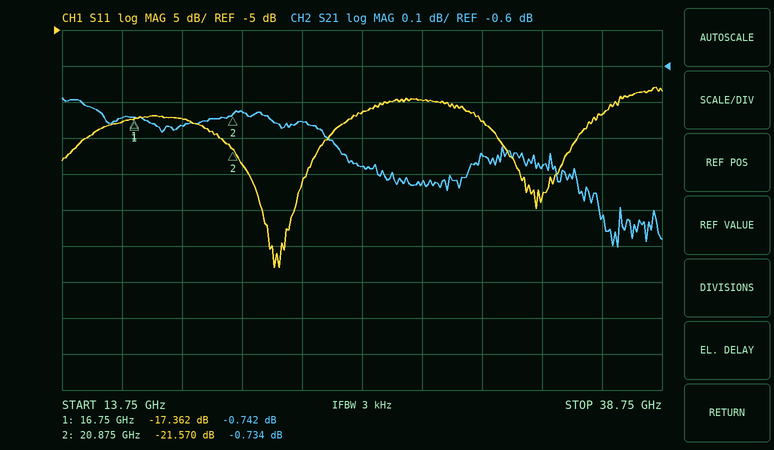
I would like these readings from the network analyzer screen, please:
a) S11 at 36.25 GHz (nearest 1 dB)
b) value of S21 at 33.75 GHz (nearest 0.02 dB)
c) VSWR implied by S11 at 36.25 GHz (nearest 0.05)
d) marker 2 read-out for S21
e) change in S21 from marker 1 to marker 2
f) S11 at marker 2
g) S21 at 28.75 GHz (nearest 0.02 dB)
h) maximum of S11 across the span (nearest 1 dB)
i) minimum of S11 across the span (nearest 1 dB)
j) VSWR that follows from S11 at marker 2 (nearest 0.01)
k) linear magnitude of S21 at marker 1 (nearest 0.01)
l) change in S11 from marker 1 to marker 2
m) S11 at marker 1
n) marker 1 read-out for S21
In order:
-17 dB
-0.88 dB
1.35
-0.734 dB
0.008 dB
-21.570 dB
-0.92 dB
-13 dB
-38 dB
1.18
0.92
-4.208 dB
-17.362 dB
-0.742 dB
